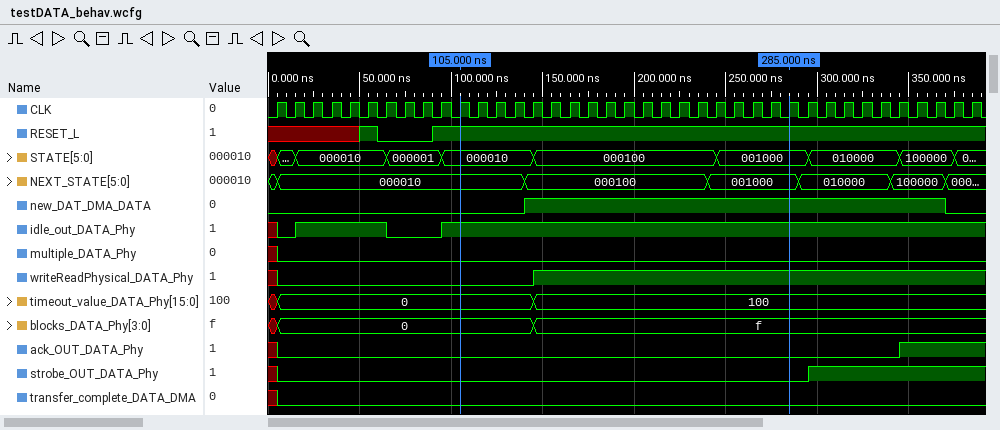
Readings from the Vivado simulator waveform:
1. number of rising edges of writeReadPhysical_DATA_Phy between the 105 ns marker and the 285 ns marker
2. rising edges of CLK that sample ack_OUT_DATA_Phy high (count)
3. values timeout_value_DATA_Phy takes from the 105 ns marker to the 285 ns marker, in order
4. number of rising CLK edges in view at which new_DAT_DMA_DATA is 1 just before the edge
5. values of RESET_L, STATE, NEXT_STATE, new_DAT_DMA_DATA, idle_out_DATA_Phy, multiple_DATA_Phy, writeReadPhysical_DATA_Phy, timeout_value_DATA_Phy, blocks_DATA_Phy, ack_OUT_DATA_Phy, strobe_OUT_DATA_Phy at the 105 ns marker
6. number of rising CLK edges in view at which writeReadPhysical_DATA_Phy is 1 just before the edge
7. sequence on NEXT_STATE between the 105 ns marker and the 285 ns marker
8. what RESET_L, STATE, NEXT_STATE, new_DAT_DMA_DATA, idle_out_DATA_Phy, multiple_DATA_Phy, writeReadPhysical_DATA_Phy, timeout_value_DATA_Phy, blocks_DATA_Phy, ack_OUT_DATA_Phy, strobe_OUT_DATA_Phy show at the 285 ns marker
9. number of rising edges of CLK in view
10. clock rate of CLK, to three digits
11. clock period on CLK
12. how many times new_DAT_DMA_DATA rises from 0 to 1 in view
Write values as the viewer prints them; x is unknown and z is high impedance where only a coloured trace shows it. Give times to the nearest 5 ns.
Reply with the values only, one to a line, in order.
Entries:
1
4
0, 100
23
RESET_L=1, STATE=000010, NEXT_STATE=000010, new_DAT_DMA_DATA=0, idle_out_DATA_Phy=1, multiple_DATA_Phy=0, writeReadPhysical_DATA_Phy=0, timeout_value_DATA_Phy=0, blocks_DATA_Phy=0, ack_OUT_DATA_Phy=0, strobe_OUT_DATA_Phy=0
24
000010, 000100, 001000
RESET_L=1, STATE=001000, NEXT_STATE=001000, new_DAT_DMA_DATA=1, idle_out_DATA_Phy=1, multiple_DATA_Phy=0, writeReadPhysical_DATA_Phy=1, timeout_value_DATA_Phy=100, blocks_DATA_Phy=f, ack_OUT_DATA_Phy=0, strobe_OUT_DATA_Phy=0
39
100 MHz
10 ns
1
